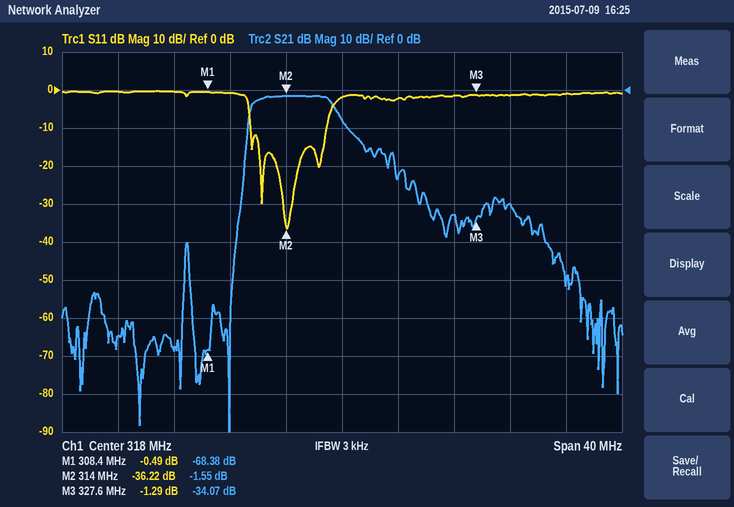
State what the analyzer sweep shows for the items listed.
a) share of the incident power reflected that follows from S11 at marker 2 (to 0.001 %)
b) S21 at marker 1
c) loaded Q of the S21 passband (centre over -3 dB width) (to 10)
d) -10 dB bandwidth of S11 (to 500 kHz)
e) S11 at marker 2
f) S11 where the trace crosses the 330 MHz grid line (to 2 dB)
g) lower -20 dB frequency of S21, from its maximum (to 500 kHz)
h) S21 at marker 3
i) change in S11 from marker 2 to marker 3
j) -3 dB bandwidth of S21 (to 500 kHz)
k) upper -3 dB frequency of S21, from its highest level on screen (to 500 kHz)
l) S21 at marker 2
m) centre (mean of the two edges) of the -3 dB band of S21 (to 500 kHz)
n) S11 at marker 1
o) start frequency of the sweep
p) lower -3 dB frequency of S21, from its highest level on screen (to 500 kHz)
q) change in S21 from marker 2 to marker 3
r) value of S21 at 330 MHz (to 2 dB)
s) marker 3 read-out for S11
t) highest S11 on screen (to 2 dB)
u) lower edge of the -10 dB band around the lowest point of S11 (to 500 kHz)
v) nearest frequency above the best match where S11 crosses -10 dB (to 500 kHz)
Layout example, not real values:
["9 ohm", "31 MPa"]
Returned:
["0.024 %", "-68.38 dB", "50", "5.5 MHz", "-36.22 dB", "-2 dB", "311.0 MHz", "-34.07 dB", "34.93 dB", "6.0 MHz", "317.5 MHz", "-1.55 dB", "314.5 MHz", "-0.49 dB", "298 MHz", "311.5 MHz", "-32.52 dB", "-30 dB", "-1.29 dB", "0 dB", "311.5 MHz", "317.0 MHz"]
